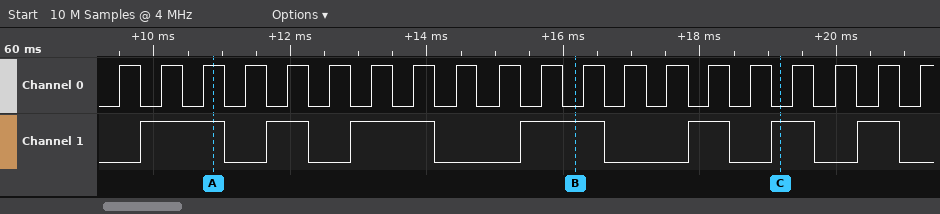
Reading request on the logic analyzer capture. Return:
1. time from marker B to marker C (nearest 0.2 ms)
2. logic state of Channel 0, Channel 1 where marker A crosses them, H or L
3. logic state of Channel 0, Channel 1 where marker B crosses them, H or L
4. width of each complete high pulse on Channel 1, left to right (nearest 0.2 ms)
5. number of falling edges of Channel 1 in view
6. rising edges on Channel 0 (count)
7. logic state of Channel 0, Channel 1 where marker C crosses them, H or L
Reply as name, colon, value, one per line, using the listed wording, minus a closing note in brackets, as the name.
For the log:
time from marker B to marker C: 3 ms
logic state of Channel 0, Channel 1 where marker A crosses them, H or L: Channel 0=H, Channel 1=H
logic state of Channel 0, Channel 1 where marker B crosses them, H or L: Channel 0=L, Channel 1=H
width of each complete high pulse on Channel 1, left to right: 1.2 ms, 0.6 ms, 1.2 ms, 1.2 ms, 0.6 ms, 0.6 ms, 0.6 ms
number of falling edges of Channel 1 in view: 7
rising edges on Channel 0: 20
logic state of Channel 0, Channel 1 where marker C crosses them, H or L: Channel 0=L, Channel 1=H
